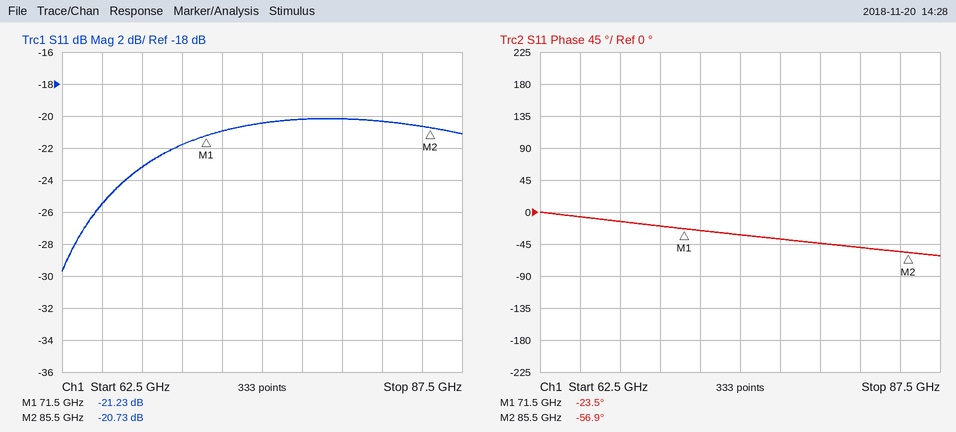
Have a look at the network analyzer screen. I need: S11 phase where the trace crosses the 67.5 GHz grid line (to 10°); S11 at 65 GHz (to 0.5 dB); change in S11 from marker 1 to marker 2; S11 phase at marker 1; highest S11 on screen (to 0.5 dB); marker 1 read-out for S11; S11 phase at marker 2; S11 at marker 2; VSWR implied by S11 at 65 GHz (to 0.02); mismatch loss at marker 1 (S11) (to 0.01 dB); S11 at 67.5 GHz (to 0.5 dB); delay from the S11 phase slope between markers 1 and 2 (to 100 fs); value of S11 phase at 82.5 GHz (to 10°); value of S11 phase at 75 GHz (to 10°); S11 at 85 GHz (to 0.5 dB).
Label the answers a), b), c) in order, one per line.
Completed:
a) -10°
b) -25.5 dB
c) 0.50 dB
d) -23.5°
e) -20.0 dB
f) -21.23 dB
g) -56.9°
h) -20.73 dB
i) 1.12
j) 0.03 dB
k) -23.0 dB
l) 6.6 ps
m) -50°
n) -30°
o) -20.5 dB
